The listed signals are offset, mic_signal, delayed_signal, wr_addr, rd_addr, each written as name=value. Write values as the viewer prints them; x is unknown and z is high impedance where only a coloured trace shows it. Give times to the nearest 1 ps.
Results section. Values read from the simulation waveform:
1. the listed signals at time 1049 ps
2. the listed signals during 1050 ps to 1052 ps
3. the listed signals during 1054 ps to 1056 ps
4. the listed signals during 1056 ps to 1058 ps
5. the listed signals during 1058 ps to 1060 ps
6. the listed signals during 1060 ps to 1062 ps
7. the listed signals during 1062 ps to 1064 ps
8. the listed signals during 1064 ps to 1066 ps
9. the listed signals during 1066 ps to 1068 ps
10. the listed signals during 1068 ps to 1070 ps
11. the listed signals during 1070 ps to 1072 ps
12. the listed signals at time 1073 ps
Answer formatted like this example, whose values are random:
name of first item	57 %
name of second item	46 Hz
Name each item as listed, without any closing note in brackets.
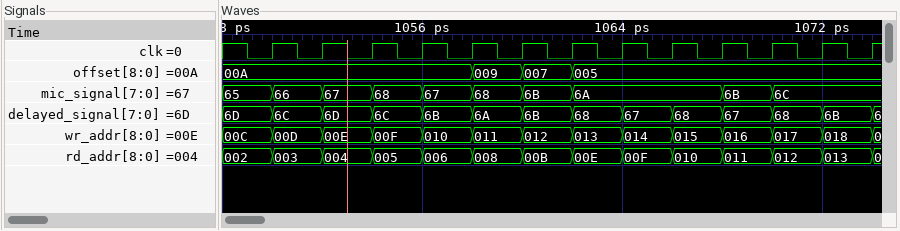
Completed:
the listed signals at time 1049 ps	offset=00A, mic_signal=65, delayed_signal=6D, wr_addr=00C, rd_addr=002
the listed signals during 1050 ps to 1052 ps	offset=00A, mic_signal=66, delayed_signal=6C, wr_addr=00D, rd_addr=003
the listed signals during 1054 ps to 1056 ps	offset=00A, mic_signal=68, delayed_signal=6C, wr_addr=00F, rd_addr=005
the listed signals during 1056 ps to 1058 ps	offset=00A, mic_signal=67, delayed_signal=6B, wr_addr=010, rd_addr=006
the listed signals during 1058 ps to 1060 ps	offset=009, mic_signal=68, delayed_signal=6A, wr_addr=011, rd_addr=008
the listed signals during 1060 ps to 1062 ps	offset=007, mic_signal=6B, delayed_signal=6B, wr_addr=012, rd_addr=00B
the listed signals during 1062 ps to 1064 ps	offset=005, mic_signal=6A, delayed_signal=68, wr_addr=013, rd_addr=00E
the listed signals during 1064 ps to 1066 ps	offset=005, mic_signal=6A, delayed_signal=67, wr_addr=014, rd_addr=00F
the listed signals during 1066 ps to 1068 ps	offset=005, mic_signal=6A, delayed_signal=68, wr_addr=015, rd_addr=010
the listed signals during 1068 ps to 1070 ps	offset=005, mic_signal=6B, delayed_signal=67, wr_addr=016, rd_addr=011
the listed signals during 1070 ps to 1072 ps	offset=005, mic_signal=6C, delayed_signal=68, wr_addr=017, rd_addr=012
the listed signals at time 1073 ps	offset=005, mic_signal=6C, delayed_signal=6B, wr_addr=018, rd_addr=013
